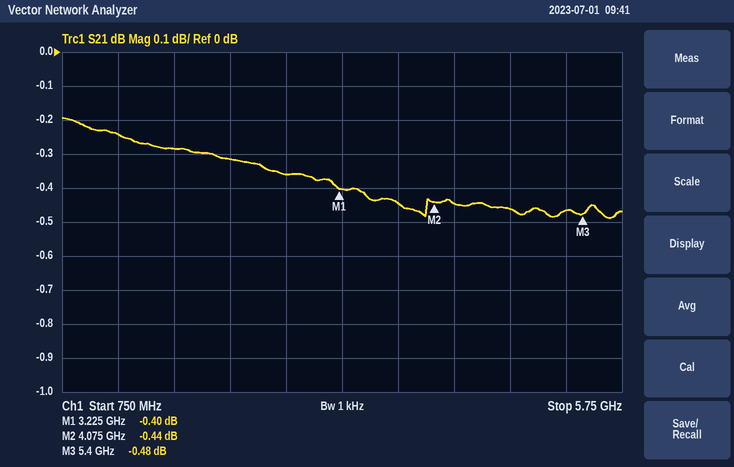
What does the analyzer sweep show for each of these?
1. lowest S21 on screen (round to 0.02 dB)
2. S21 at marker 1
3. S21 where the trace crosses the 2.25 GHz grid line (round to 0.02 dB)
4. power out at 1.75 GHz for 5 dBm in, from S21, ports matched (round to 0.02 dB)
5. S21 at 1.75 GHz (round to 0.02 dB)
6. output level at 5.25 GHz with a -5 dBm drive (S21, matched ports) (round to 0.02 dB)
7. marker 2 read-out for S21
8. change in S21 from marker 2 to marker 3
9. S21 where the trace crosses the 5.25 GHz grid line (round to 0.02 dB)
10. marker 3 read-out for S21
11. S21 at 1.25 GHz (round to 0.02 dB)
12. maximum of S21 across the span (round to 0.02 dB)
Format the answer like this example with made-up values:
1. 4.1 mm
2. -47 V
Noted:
1. -0.48 dB
2. -0.40 dB
3. -0.32 dB
4. 4.72 dBm
5. -0.28 dB
6. -5.46 dBm
7. -0.44 dB
8. -0.04 dB
9. -0.46 dB
10. -0.48 dB
11. -0.24 dB
12. -0.20 dB
